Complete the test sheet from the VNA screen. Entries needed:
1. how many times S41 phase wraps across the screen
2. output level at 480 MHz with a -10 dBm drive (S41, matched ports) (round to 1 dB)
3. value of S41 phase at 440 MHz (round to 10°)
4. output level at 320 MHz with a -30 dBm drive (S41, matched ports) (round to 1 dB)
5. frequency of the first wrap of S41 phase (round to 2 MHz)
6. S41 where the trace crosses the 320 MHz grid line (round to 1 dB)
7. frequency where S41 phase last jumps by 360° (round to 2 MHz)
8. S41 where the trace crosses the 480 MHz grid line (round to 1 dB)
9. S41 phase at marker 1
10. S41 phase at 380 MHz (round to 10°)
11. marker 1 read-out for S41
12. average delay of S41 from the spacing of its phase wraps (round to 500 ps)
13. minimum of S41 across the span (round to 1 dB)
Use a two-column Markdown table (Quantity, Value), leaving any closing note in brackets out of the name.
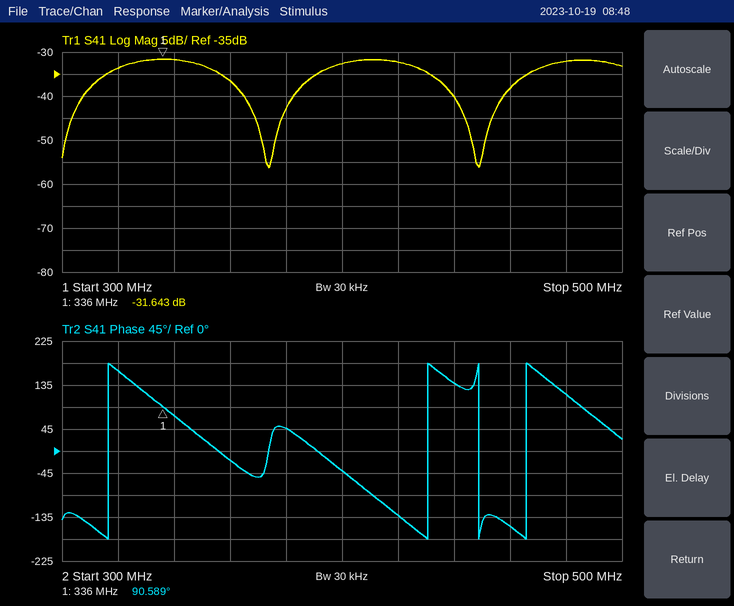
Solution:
| Quantity | Value |
|---|---|
| how many times S41 phase wraps across the screen | 4 |
| output level at 480 MHz with a -10 dBm drive (S41, matched ports) | -42 dBm |
| value of S41 phase at 440 MHz | 140° |
| output level at 320 MHz with a -30 dBm drive (S41, matched ports) | -64 dBm |
| frequency of the first wrap of S41 phase | 316 MHz |
| S41 where the trace crosses the 320 MHz grid line | -34 dB |
| frequency where S41 phase last jumps by 360° | 466 MHz |
| S41 where the trace crosses the 480 MHz grid line | -32 dB |
| S41 phase at marker 1 | 90.589° |
| S41 phase at 380 MHz | 50° |
| marker 1 read-out for S41 | -31.643 dB |
| average delay of S41 from the spacing of its phase wraps | 20.0 ns |
| minimum of S41 across the span | -56 dB |
